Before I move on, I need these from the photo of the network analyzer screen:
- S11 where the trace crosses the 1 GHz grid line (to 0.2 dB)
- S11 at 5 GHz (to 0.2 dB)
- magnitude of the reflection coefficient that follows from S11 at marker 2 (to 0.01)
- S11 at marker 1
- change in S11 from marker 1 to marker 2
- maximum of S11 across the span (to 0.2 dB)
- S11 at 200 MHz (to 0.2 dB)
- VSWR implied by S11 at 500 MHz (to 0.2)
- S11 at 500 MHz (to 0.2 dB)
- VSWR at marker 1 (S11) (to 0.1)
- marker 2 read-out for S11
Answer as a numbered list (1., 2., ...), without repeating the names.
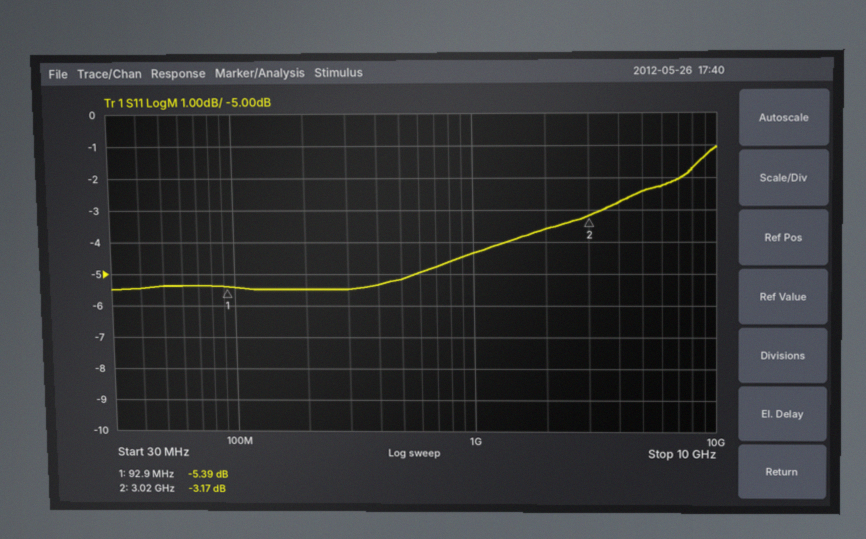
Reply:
1. -4.4 dB
2. -2.4 dB
3. 0.69
4. -5.39 dB
5. 2.22 dB
6. -1.0 dB
7. -5.4 dB
8. 3.4
9. -5.2 dB
10. 3.3
11. -3.17 dB
